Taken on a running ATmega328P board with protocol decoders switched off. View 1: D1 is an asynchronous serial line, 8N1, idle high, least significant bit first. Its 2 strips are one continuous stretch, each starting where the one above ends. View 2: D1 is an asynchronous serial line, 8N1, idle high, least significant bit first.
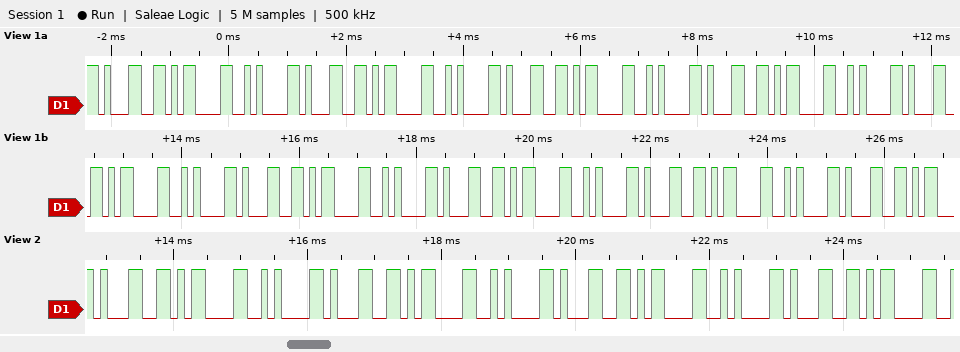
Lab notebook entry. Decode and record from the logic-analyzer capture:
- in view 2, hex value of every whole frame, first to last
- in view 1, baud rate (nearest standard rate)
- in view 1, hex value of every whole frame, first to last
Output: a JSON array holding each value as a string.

["31 0D 0A 31 0D 0A 31 0D 0A 31 0D", "9600 baud", "31 0D 0A 31 0D 0A 31 0D 0A 31 0D 0A 31 0D 0A 31 0D 0A 31 0D 0A 31 0D 0A 31"]
